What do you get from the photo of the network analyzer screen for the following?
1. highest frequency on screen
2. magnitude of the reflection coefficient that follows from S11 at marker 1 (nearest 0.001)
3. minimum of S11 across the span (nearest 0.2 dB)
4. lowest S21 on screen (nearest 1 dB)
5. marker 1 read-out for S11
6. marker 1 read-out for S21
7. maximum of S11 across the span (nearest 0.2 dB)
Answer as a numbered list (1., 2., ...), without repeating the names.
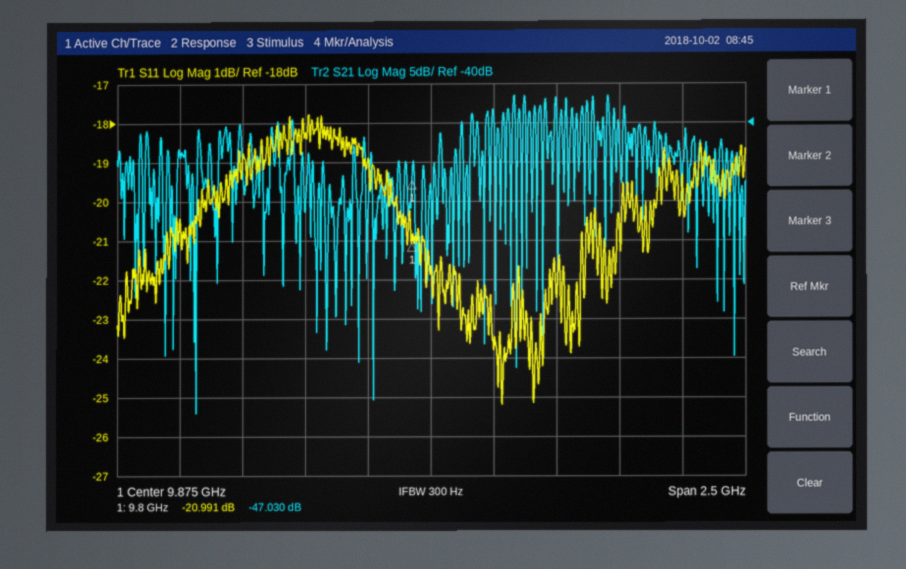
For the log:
1. 11.125 GHz
2. 0.089
3. -25.2 dB
4. -77 dB
5. -20.991 dB
6. -47.030 dB
7. -17.8 dB
